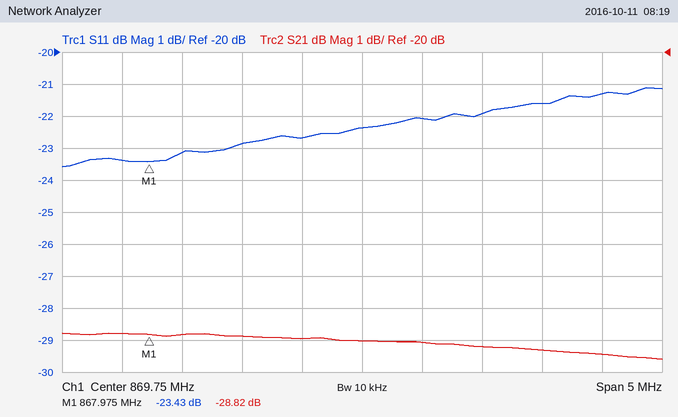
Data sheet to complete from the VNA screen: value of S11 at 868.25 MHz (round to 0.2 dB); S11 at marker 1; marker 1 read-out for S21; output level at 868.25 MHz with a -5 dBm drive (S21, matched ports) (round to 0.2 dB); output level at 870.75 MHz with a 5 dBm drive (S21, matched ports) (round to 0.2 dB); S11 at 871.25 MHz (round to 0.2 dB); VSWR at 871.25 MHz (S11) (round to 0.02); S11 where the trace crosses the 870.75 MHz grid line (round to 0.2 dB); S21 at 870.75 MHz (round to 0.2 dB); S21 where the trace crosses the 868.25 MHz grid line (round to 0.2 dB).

-23.2 dB
-23.43 dB
-28.82 dB
-33.8 dBm
-24.2 dBm
-21.6 dB
1.18
-22.0 dB
-29.2 dB
-28.8 dB
